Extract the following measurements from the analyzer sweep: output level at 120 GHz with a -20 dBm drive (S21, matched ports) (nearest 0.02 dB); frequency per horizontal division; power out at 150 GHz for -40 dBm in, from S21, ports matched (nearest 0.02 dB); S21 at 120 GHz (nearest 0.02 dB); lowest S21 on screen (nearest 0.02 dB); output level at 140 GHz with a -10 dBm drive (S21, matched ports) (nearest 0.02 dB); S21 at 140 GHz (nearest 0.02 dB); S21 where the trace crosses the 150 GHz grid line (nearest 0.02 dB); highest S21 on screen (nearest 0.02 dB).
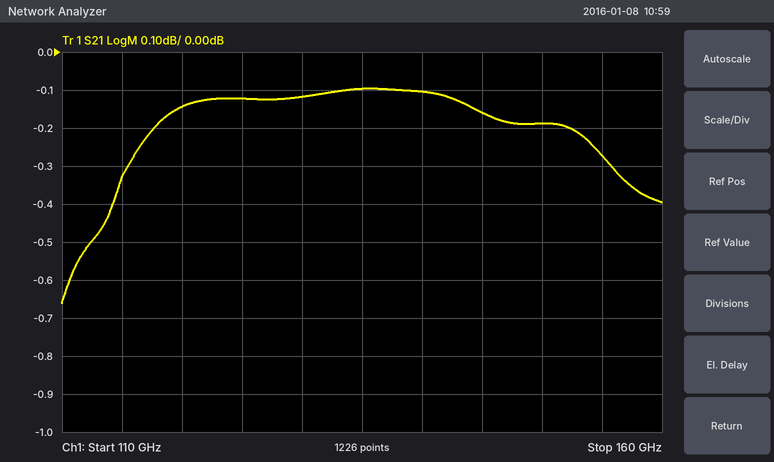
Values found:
-20.14 dBm
5 GHz
-40.18 dBm
-0.14 dB
-0.66 dB
-10.10 dBm
-0.10 dB
-0.18 dB
-0.10 dB
